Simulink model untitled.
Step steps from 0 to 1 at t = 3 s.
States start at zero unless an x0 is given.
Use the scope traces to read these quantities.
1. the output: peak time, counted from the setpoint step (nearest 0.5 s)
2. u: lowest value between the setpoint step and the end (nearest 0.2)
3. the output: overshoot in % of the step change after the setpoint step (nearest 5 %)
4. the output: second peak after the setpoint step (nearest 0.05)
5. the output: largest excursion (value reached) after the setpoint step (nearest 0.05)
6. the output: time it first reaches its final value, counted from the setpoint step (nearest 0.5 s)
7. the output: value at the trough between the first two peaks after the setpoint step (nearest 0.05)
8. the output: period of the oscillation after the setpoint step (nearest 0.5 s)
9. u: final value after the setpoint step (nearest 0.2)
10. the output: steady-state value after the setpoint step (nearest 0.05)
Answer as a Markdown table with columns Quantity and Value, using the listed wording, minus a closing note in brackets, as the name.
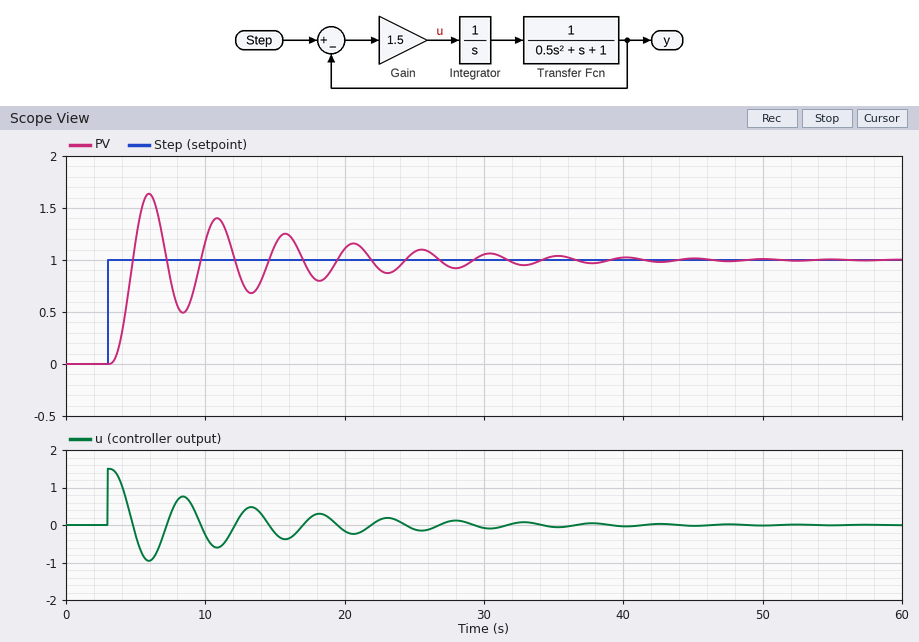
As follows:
| Quantity | Value |
|---|---|
| the output: peak time, counted from the setpoint step | 3.0 s |
| u: lowest value between the setpoint step and the end | -1.0 |
| the output: overshoot in % of the step change after the setpoint step | 65 % |
| the output: second peak after the setpoint step | 1.40 |
| the output: largest excursion (value reached) after the setpoint step | 1.65 |
| the output: time it first reaches its final value, counted from the setpoint step | 2.0 s |
| the output: value at the trough between the first two peaks after the setpoint step | 0.50 |
| the output: period of the oscillation after the setpoint step | 5.0 s |
| u: final value after the setpoint step | 0.0 |
| the output: steady-state value after the setpoint step | 1.00 |
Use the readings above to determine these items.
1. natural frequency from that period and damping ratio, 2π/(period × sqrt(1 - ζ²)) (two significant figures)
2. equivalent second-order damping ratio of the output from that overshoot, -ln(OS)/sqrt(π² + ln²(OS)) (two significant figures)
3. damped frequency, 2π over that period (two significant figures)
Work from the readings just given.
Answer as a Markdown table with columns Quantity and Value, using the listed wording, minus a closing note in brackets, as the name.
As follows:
| Quantity | Value |
|---|---|
| natural frequency from that period and damping ratio, 2π/(period × sqrt(1 - ζ²)) | 1.3 rad/s |
| equivalent second-order damping ratio of the output from that overshoot, -ln(OS)/sqrt(π² + ln²(OS)) | 0.14 |
| damped frequency, 2π over that period | 1.3 rad/s |
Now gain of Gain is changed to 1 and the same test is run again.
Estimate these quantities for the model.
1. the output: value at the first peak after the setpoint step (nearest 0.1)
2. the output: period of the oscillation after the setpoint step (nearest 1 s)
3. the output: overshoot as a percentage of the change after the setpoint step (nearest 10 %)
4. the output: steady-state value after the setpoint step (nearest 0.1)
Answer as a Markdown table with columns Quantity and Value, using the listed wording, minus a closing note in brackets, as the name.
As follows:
| Quantity | Value |
|---|---|
| the output: value at the first peak after the setpoint step | 1.4 |
| the output: period of the oscillation after the setpoint step | 6 s |
| the output: overshoot as a percentage of the change after the setpoint step | 40 % |
| the output: steady-state value after the setpoint step | 1.0 |
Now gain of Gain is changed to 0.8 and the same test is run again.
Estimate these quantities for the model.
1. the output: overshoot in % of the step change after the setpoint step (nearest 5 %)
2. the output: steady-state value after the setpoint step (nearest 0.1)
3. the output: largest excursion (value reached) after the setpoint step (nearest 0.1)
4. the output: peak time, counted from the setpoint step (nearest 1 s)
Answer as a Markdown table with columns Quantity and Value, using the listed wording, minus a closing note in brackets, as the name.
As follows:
| Quantity | Value |
|---|---|
| the output: overshoot in % of the step change after the setpoint step | 30 % |
| the output: steady-state value after the setpoint step | 1.0 |
| the output: largest excursion (value reached) after the setpoint step | 1.3 |
| the output: peak time, counted from the setpoint step | 4 s |
